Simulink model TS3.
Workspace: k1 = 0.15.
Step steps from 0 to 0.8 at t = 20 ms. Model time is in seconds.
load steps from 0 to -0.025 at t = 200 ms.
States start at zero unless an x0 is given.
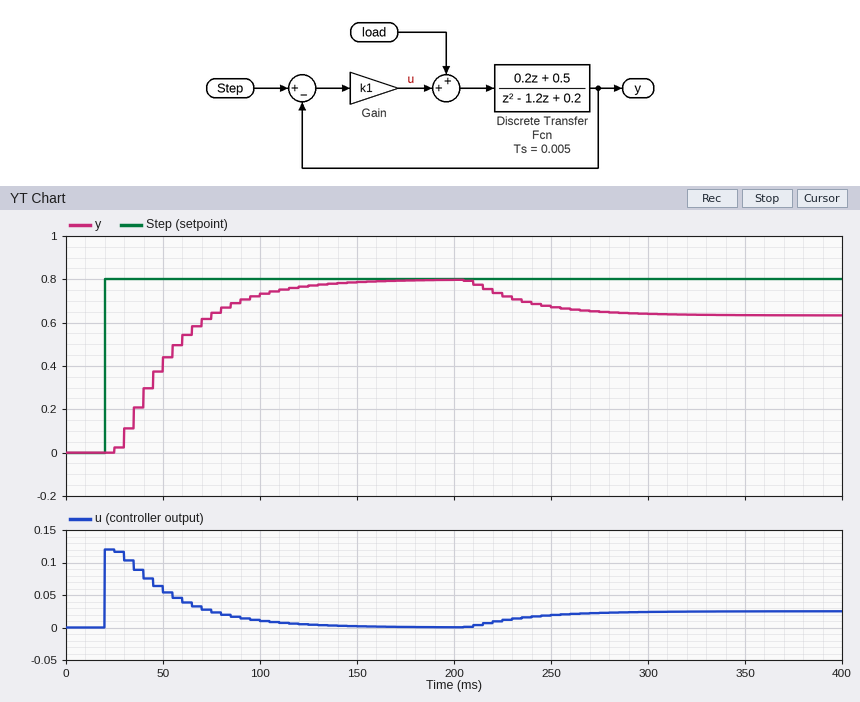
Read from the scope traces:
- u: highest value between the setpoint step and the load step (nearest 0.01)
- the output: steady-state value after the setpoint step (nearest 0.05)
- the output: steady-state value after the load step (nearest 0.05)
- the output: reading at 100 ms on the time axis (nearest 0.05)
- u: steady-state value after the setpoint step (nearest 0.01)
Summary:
0.12
0.80
0.65
0.75
0.00
